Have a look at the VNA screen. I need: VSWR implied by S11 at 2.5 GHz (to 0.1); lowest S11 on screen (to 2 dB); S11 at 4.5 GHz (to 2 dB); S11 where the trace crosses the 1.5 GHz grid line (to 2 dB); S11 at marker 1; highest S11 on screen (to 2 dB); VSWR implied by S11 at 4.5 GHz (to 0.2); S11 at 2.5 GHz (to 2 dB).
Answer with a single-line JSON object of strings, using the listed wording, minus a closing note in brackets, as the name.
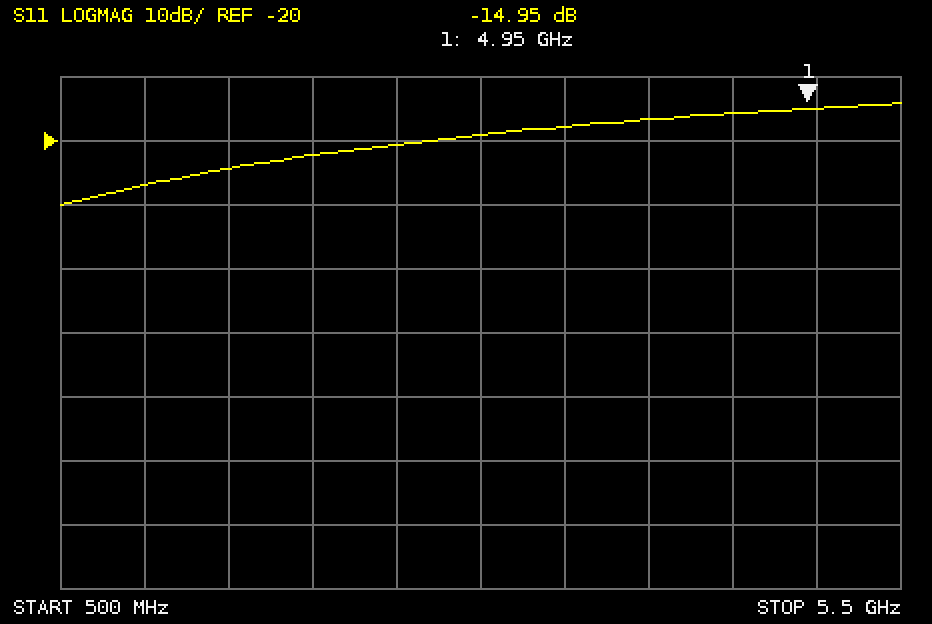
{"VSWR implied by S11 at 2.5 GHz": "1.2", "lowest S11 on screen": "-30 dB", "S11 at 4.5 GHz": "-16 dB", "S11 where the trace crosses the 1.5 GHz grid line": "-24 dB", "S11 at marker 1": "-14.95 dB", "highest S11 on screen": "-14 dB", "VSWR implied by S11 at 4.5 GHz": "1.4", "S11 at 2.5 GHz": "-20 dB"}
